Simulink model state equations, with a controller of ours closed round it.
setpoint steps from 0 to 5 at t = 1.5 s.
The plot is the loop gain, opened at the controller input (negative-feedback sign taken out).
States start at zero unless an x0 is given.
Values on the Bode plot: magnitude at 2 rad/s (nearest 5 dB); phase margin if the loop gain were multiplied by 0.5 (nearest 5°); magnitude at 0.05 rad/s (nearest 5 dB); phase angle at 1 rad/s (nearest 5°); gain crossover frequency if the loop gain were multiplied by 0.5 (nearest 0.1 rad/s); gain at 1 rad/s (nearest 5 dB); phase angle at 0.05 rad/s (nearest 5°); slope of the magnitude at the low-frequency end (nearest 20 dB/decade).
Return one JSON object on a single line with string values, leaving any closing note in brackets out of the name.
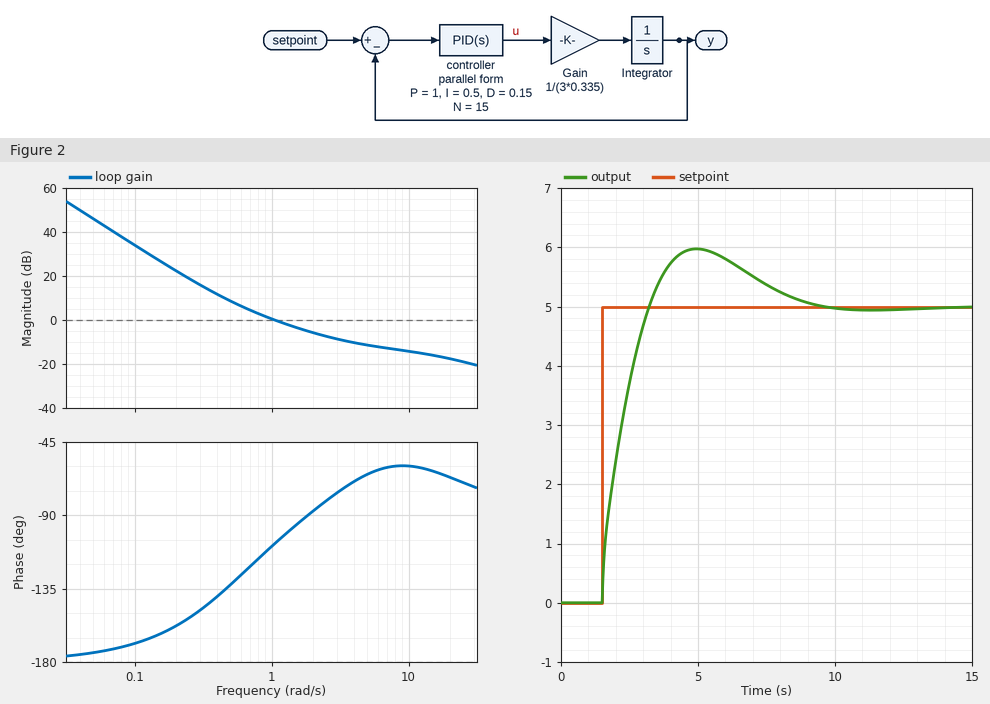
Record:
{"magnitude at 2 rad/s": "-5 dB", "phase margin if the loop gain were multiplied by 0.5": "55°", "magnitude at 0.05 rad/s": "45 dB", "phase angle at 1 rad/s": "-110°", "gain crossover frequency if the loop gain were multiplied by 0.5": "0.6 rad/s", "gain at 1 rad/s": "0 dB", "phase angle at 0.05 rad/s": "-175°", "slope of the magnitude at the low-frequency end": "-40 dB/decade"}
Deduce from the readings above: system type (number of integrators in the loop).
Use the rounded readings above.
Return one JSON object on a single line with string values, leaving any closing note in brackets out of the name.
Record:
{"system type": "2"}
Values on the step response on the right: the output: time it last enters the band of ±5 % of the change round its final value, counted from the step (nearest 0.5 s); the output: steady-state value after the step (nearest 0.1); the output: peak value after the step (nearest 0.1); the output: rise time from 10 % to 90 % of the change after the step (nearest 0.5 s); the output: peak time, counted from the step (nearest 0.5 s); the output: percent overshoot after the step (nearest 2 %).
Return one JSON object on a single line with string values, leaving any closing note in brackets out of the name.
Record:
{"the output: time it last enters the band of ±5 % of the change round its final value, counted from the step": "6.5 s", "the output: steady-state value after the step": "5.0", "the output: peak value after the step": "6.0", "the output: rise time from 10 % to 90 % of the change after the step": "1.5 s", "the output: peak time, counted from the step": "3.5 s", "the output: percent overshoot after the step": "20 %"}
